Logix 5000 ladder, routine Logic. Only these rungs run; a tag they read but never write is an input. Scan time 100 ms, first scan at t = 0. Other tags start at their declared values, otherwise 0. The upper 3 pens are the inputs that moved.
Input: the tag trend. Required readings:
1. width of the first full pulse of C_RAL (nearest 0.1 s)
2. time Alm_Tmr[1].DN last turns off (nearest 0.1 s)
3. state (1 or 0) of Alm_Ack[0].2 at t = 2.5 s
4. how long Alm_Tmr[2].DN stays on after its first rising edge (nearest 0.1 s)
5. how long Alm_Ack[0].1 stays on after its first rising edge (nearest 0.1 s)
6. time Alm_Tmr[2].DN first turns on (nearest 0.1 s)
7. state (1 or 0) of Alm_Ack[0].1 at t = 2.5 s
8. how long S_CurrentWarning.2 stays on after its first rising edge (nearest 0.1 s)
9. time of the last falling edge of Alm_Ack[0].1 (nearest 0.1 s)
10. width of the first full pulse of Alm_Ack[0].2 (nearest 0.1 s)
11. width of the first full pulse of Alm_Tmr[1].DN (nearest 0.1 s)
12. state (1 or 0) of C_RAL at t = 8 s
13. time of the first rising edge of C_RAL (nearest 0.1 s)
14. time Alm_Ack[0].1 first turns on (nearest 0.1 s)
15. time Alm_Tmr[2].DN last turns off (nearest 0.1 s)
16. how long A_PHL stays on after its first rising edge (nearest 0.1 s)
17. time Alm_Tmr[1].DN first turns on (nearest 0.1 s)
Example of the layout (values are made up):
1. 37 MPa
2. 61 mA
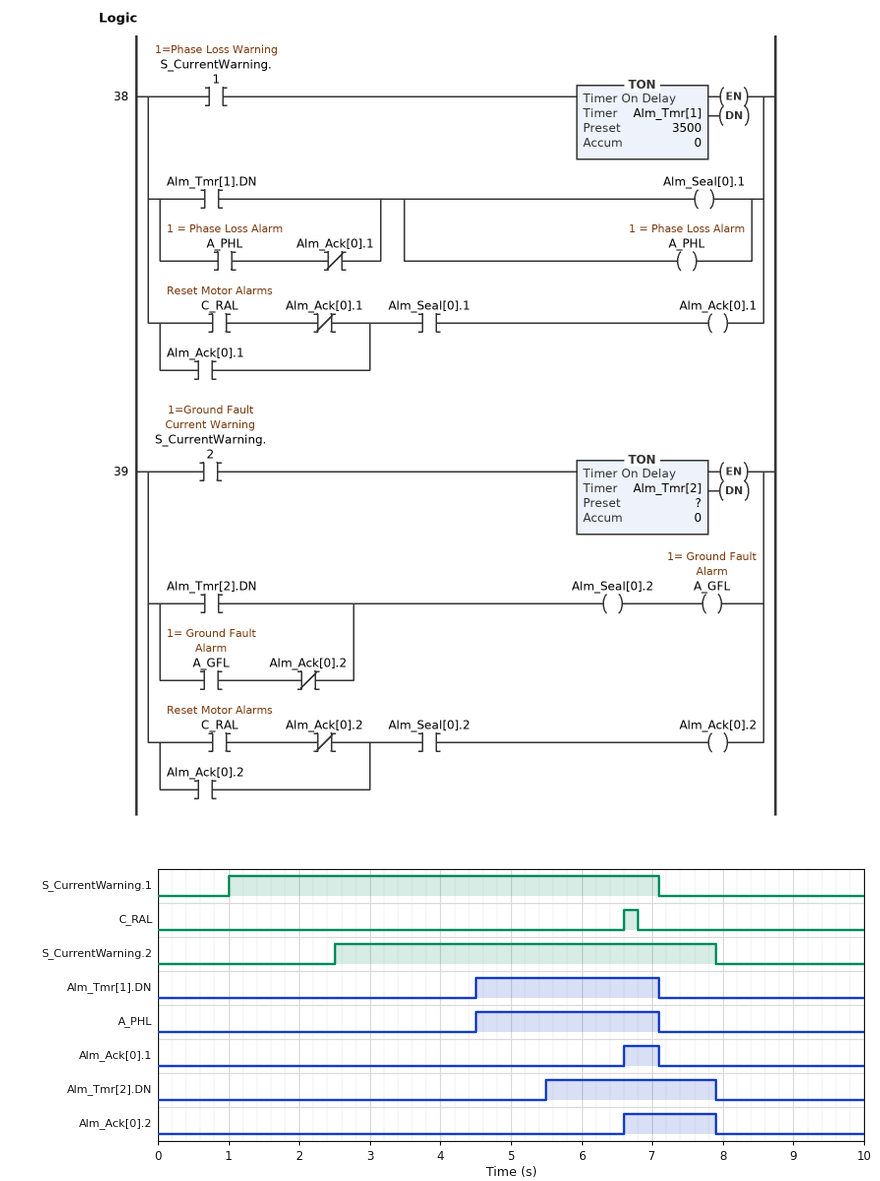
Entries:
1. 0.2 s
2. 7.1 s
3. 0
4. 2.4 s
5. 0.5 s
6. 5.5 s
7. 0
8. 5.4 s
9. 7.1 s
10. 1.3 s
11. 2.6 s
12. 0
13. 6.6 s
14. 6.6 s
15. 7.9 s
16. 2.6 s
17. 4.5 s
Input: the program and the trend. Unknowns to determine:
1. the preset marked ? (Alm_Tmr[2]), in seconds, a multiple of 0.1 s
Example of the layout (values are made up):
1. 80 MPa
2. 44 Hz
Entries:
1. 3.0 s
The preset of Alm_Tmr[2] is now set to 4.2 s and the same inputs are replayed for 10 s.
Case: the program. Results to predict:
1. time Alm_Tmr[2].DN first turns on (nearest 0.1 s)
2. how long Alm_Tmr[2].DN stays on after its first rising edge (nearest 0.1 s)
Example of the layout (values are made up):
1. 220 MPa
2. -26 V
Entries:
1. 6.7 s
2. 1.2 s
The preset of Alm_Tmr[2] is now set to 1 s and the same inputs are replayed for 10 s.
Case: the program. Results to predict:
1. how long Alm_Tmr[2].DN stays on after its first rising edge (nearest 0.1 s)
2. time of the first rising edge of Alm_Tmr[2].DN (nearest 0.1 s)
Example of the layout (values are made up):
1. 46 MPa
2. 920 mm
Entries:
1. 4.4 s
2. 3.5 s
